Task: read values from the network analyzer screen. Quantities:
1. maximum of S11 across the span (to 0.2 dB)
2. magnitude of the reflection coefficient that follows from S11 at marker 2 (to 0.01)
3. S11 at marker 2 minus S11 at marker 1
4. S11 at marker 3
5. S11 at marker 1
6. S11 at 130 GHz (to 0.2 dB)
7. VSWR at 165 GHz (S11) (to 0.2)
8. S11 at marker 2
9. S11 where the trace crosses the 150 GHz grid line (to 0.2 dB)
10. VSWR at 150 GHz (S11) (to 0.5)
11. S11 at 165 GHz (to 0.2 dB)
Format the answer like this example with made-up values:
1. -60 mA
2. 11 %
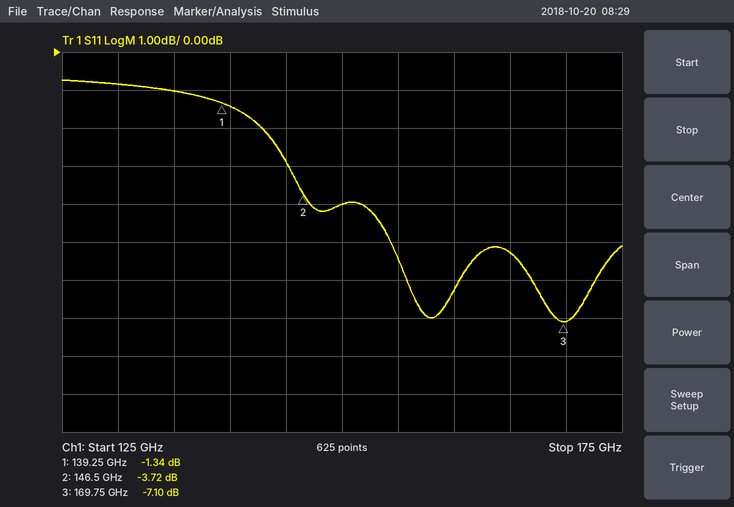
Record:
1. -0.8 dB
2. 0.65
3. -2.38 dB
4. -7.10 dB
5. -1.34 dB
6. -0.8 dB
7. 3.4
8. -3.72 dB
9. -4.0 dB
10. 4.5
11. -5.2 dB
